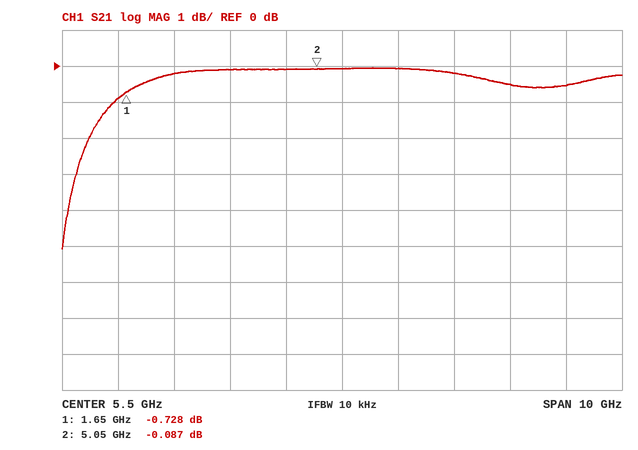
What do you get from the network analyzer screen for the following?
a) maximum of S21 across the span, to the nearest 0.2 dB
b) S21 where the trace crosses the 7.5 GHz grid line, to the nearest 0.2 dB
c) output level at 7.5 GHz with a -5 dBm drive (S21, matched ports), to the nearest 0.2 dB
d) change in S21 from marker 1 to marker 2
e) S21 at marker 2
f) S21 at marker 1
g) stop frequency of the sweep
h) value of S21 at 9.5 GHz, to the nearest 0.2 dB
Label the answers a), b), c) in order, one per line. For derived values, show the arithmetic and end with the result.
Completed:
a) 0.0 dB
b) -0.2 dB
c) -5 dBm + (-0.2 dB) = -5.2 dBm
d) -0.087 − (-0.728) = 0.641 dB
e) -0.087 dB
f) -0.728 dB
g) 10.5 GHz
h) -0.6 dB
